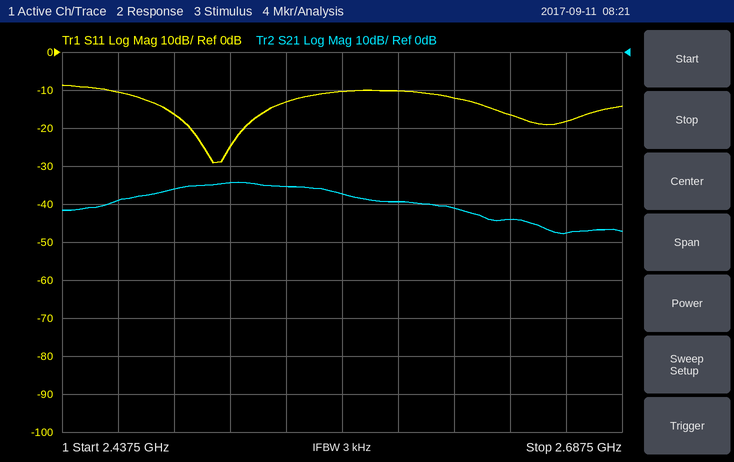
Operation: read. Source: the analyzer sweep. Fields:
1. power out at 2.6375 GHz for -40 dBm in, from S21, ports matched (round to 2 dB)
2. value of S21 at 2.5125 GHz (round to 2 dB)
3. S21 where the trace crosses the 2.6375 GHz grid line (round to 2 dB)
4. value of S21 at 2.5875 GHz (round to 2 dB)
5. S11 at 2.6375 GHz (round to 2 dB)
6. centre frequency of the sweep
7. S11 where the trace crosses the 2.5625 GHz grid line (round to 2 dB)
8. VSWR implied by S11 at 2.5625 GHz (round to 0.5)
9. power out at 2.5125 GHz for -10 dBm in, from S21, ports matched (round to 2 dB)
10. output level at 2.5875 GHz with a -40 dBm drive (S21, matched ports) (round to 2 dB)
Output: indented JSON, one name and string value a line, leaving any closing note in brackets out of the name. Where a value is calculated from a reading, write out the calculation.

{
  "power out at 2.6375 GHz for -40 dBm in, from S21, ports matched": "-40 dBm + (-44 dB) = -84 dBm",
  "value of S21 at 2.5125 GHz": "-34 dB",
  "S21 where the trace crosses the 2.6375 GHz grid line": "-44 dB",
  "value of S21 at 2.5875 GHz": "-40 dB",
  "S11 at 2.6375 GHz": "-16 dB",
  "centre frequency of the sweep": "2.5625 GHz",
  "S11 where the trace crosses the 2.5625 GHz grid line": "-10 dB",
  "VSWR implied by S11 at 2.5625 GHz": "|Γ| = 10^(-10/20) = 0.3162; VSWR = (1 + 0.3162)/(1 − 0.3162) ≈ 1.92, so 2.0 to the nearest 0.5",
  "power out at 2.5125 GHz for -10 dBm in, from S21, ports matched": "-10 dBm + (-34 dB) = -44 dBm",
  "output level at 2.5875 GHz with a -40 dBm drive (S21, matched ports)": "-40 dBm + (-40 dB) = -80 dBm"
}
